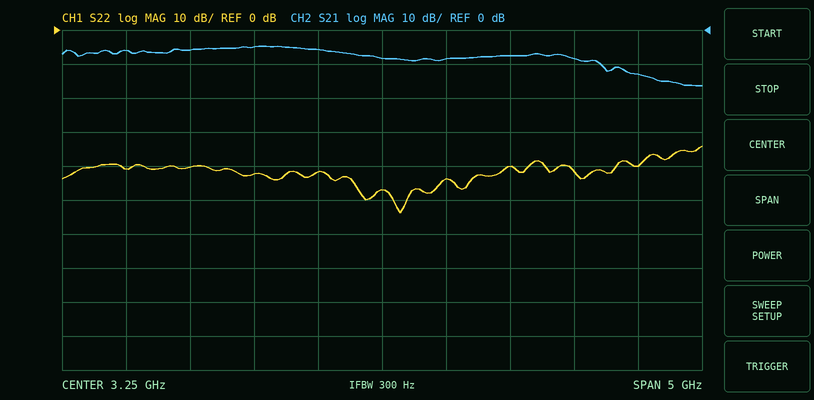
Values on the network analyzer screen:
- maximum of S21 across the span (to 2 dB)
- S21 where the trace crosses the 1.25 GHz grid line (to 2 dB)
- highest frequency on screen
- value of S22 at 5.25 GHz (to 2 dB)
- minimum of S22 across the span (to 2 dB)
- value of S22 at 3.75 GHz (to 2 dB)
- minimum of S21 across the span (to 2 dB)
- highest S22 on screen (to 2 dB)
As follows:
-4 dB
-6 dB
5.75 GHz
-40 dB
-54 dB
-44 dB
-16 dB
-34 dB
